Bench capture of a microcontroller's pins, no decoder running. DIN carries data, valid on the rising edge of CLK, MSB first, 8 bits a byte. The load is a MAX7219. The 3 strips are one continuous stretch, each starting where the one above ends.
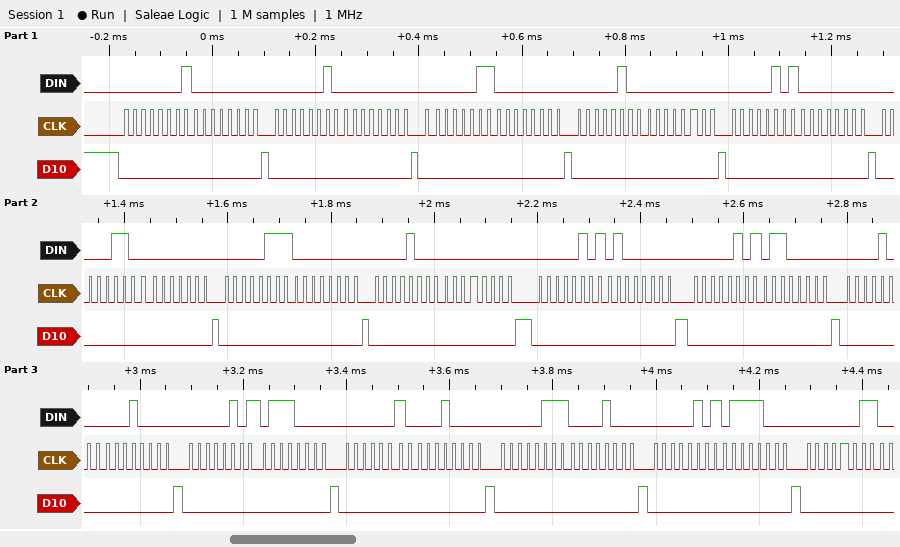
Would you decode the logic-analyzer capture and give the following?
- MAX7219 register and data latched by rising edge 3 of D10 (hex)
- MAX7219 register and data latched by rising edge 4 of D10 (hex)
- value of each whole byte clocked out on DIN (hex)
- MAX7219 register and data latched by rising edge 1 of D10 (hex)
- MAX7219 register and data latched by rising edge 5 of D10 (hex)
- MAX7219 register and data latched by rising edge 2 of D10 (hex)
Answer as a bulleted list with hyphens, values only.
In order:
- register 0x3, data 0x00
- register 0x4, data 0x00
- 01 00 02 00 03 00 04 00 05 00 06 00 07 00 08 00 05 40 05 60 08 10 05 70 02 10 07 08 05 78 03
- register 0x1, data 0x00
- register 0x5, data 0x00
- register 0x2, data 0x00
